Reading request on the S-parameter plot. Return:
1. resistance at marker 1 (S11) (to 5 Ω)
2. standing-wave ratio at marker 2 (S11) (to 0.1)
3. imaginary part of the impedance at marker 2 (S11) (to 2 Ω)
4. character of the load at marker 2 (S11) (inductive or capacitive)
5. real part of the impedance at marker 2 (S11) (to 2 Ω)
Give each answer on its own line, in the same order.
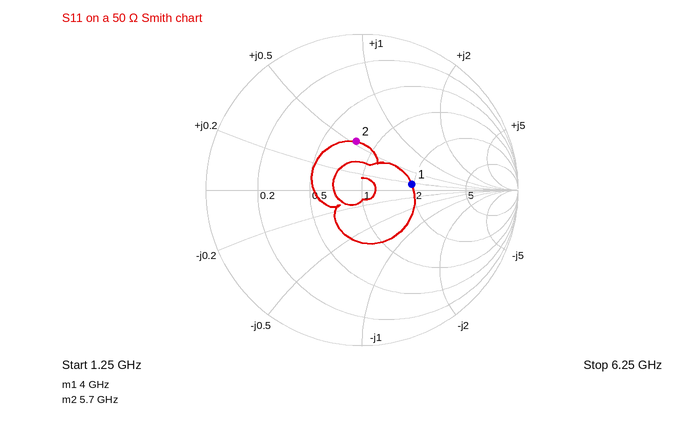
95 Ω
1.9
+26 Ω
inductive
38 Ω
